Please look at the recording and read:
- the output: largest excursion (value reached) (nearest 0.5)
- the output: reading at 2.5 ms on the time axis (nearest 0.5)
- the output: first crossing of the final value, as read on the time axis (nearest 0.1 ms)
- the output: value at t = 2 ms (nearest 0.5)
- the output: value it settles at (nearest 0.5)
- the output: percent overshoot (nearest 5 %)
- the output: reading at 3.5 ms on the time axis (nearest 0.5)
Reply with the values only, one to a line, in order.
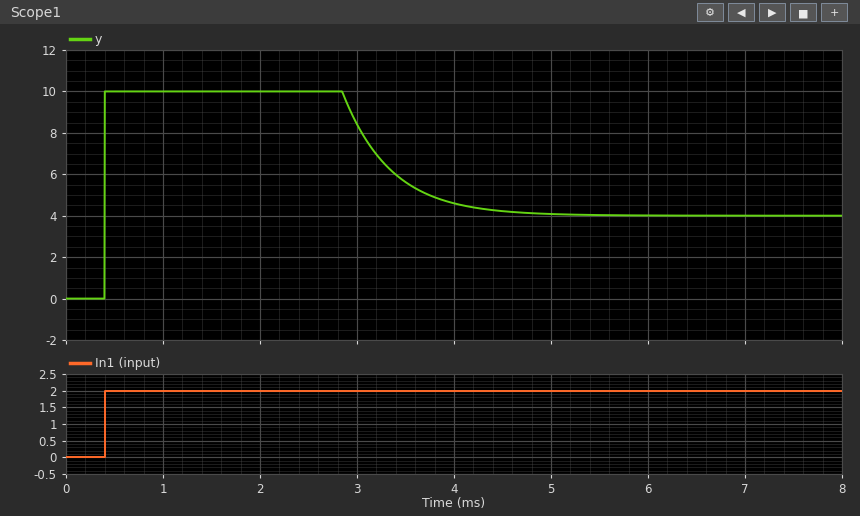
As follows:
10.0
10.0
0.4 ms
10.0
4.0
150 %
5.5
